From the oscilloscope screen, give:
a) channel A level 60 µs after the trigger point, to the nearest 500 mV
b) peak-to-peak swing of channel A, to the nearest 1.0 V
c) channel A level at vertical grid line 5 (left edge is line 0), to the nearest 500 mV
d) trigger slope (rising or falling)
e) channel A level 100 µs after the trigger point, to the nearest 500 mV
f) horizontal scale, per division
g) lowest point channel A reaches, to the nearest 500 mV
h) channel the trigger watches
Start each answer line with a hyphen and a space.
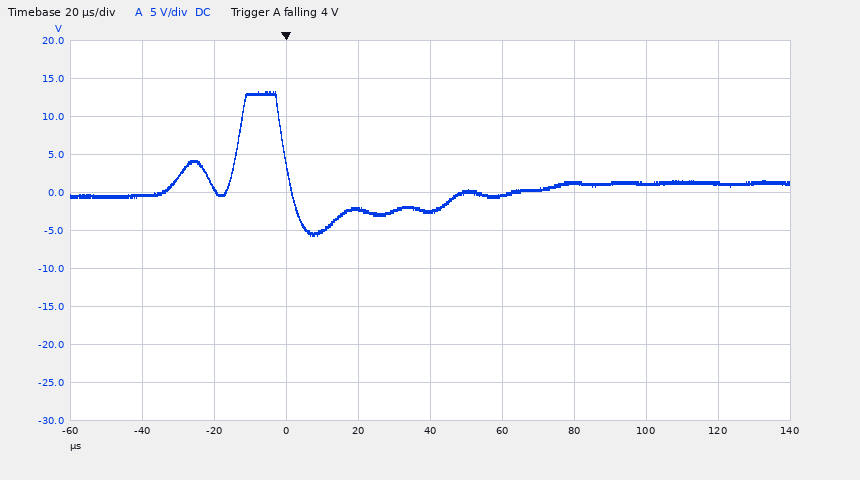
- -500 mV
- 19.0 V
- -2.5 V
- falling
- 1.0 V
- 20 µs
- -5.5 V
- channel A
